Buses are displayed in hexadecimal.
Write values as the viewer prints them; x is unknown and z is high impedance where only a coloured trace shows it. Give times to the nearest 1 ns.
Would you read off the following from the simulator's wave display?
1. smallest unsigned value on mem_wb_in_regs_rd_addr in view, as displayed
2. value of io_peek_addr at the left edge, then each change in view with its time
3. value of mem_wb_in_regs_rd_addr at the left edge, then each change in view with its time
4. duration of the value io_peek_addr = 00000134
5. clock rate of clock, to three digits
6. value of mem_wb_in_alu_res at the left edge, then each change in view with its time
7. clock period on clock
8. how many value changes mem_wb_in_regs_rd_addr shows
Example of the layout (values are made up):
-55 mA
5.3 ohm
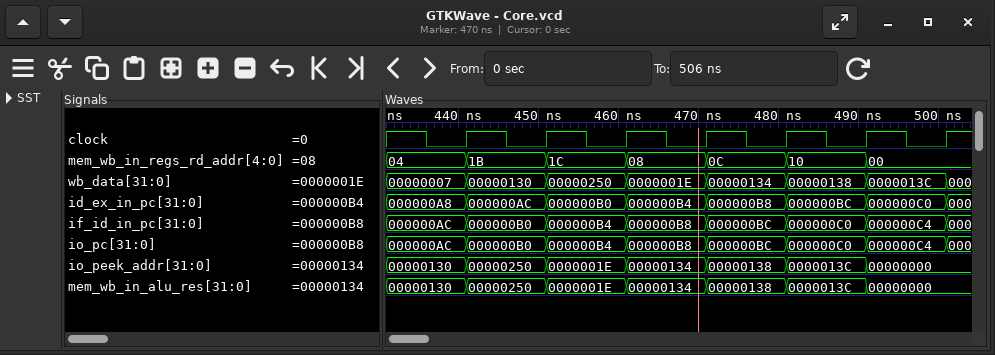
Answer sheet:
00
00000130, 00000250 at 441 ns, 0000001E at 451 ns, 00000134 at 461 ns, 00000138 at 471 ns, 0000013C at 481 ns, 00000000 at 491 ns
04, 1B at 441 ns, 1C at 451 ns, 08 at 461 ns, 0C at 471 ns, 10 at 481 ns, 00 at 491 ns
10 ns
100 MHz
00000130, 00000250 at 441 ns, 0000001E at 451 ns, 00000134 at 461 ns, 00000138 at 471 ns, 0000013C at 481 ns, 00000000 at 491 ns
10 ns
6
